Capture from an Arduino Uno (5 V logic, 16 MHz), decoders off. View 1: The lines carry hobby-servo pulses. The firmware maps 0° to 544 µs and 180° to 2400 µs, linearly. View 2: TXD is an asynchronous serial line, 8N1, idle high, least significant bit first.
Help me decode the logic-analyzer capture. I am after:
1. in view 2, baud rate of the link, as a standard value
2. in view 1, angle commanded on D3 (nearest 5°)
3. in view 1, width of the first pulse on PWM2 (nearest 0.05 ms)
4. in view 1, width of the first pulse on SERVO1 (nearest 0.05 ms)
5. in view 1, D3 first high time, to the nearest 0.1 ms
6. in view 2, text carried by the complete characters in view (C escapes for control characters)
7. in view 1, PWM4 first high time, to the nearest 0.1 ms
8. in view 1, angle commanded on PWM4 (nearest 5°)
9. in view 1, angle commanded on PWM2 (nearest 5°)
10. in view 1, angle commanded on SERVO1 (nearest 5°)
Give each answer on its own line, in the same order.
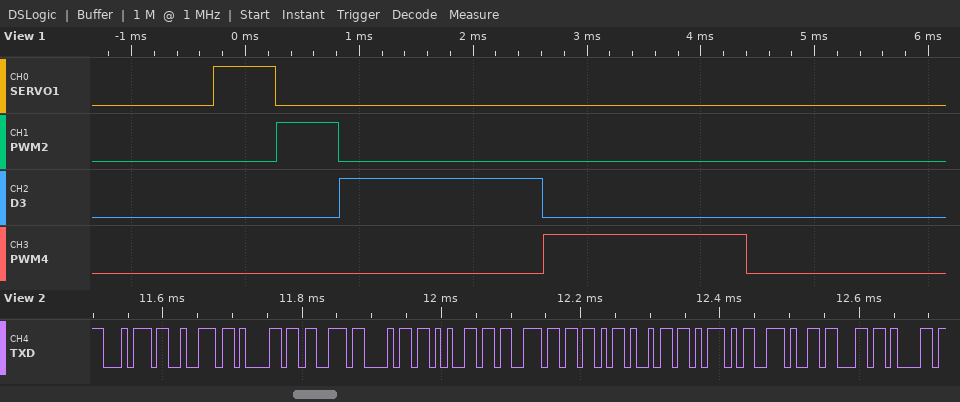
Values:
115200 baud
120°
0.55 ms
0.55 ms
1.8 ms
"trashes[i].ca"
1.8 ms
120°
0°
0°
